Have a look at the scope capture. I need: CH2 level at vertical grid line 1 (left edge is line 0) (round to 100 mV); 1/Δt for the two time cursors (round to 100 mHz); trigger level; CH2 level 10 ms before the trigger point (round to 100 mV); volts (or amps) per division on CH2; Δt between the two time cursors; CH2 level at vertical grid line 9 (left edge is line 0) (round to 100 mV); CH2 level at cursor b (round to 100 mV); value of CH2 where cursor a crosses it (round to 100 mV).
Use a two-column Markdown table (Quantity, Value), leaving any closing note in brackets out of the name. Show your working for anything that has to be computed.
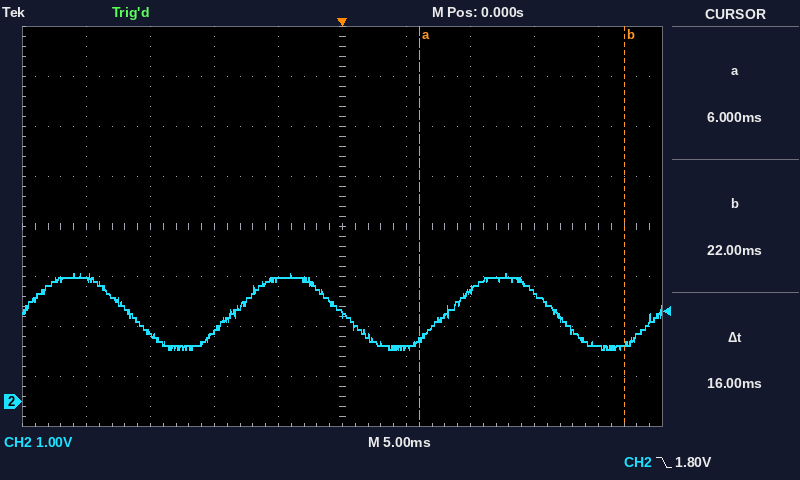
| Quantity | Value |
|---|---|
| CH2 level at vertical grid line 1 (left edge is line 0) | 2.4 V |
| 1/Δt for the two time cursors | 1 / 16 ms ≈ 62.5 Hz |
| trigger level | 1.80 V |
| CH2 level 10 ms before the trigger point | 1.4 V |
| volts (or amps) per division on CH2 | 1 V |
| Δt between the two time cursors | 16 ms |
| CH2 level at vertical grid line 9 (left edge is line 0) | 1.1 V |
| CH2 level at cursor b | 1.2 V |
| value of CH2 where cursor a crosses it | 1.3 V |
